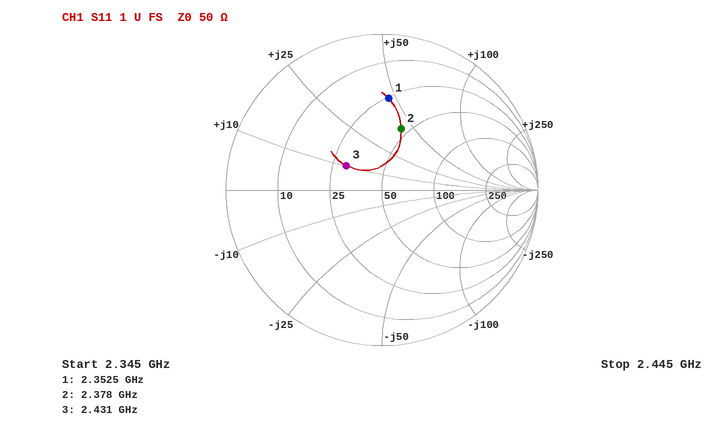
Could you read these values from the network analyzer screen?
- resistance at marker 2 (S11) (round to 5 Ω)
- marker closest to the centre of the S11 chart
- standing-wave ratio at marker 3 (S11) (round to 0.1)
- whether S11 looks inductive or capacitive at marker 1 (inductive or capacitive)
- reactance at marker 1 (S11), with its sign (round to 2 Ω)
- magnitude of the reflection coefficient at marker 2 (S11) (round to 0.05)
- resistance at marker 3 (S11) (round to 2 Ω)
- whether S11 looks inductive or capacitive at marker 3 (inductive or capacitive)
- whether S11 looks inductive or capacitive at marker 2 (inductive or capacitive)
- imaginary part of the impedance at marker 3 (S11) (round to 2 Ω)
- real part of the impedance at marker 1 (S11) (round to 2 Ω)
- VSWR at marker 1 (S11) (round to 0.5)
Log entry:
45 Ω
marker 3
1.8
inductive
+46 Ω
0.40
30 Ω
inductive
inductive
+10 Ω
26 Ω
4.0
